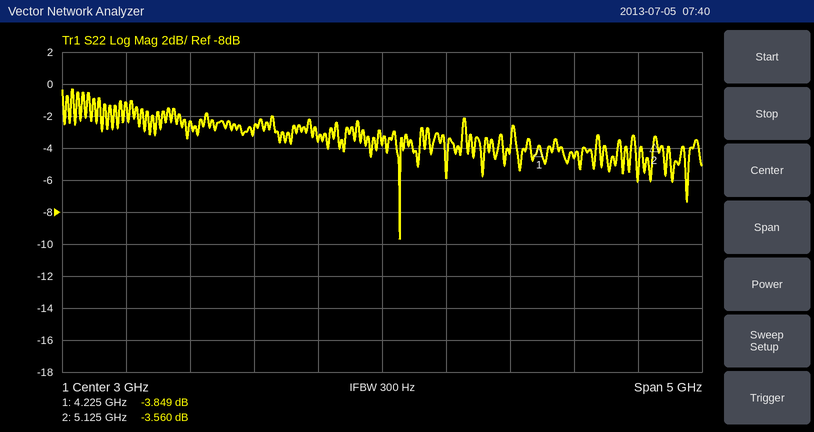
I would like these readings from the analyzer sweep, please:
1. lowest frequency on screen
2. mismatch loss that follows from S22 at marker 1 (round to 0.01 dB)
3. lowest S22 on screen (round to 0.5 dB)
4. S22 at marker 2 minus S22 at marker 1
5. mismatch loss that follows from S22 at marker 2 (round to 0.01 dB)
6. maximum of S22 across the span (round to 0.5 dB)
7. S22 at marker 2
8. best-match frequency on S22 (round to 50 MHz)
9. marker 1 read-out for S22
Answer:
500 MHz
2.31 dB
-9.5 dB
0.289 dB
2.52 dB
-0.5 dB
-3.560 dB
3.15 GHz
-3.849 dB
